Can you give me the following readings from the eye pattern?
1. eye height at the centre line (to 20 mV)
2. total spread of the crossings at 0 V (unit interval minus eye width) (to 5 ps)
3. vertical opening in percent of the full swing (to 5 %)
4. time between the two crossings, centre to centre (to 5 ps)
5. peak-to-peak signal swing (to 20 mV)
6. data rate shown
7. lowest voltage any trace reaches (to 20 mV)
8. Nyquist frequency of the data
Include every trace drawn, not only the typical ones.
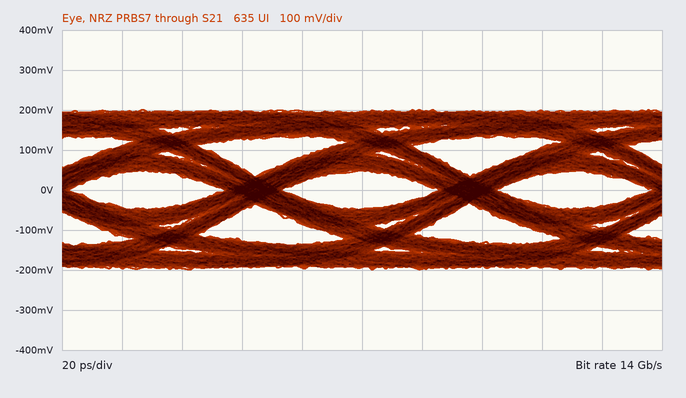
100 mV
20 ps
25 %
70 ps
400 mV
14 Gb/s
-200 mV
7 GHz
